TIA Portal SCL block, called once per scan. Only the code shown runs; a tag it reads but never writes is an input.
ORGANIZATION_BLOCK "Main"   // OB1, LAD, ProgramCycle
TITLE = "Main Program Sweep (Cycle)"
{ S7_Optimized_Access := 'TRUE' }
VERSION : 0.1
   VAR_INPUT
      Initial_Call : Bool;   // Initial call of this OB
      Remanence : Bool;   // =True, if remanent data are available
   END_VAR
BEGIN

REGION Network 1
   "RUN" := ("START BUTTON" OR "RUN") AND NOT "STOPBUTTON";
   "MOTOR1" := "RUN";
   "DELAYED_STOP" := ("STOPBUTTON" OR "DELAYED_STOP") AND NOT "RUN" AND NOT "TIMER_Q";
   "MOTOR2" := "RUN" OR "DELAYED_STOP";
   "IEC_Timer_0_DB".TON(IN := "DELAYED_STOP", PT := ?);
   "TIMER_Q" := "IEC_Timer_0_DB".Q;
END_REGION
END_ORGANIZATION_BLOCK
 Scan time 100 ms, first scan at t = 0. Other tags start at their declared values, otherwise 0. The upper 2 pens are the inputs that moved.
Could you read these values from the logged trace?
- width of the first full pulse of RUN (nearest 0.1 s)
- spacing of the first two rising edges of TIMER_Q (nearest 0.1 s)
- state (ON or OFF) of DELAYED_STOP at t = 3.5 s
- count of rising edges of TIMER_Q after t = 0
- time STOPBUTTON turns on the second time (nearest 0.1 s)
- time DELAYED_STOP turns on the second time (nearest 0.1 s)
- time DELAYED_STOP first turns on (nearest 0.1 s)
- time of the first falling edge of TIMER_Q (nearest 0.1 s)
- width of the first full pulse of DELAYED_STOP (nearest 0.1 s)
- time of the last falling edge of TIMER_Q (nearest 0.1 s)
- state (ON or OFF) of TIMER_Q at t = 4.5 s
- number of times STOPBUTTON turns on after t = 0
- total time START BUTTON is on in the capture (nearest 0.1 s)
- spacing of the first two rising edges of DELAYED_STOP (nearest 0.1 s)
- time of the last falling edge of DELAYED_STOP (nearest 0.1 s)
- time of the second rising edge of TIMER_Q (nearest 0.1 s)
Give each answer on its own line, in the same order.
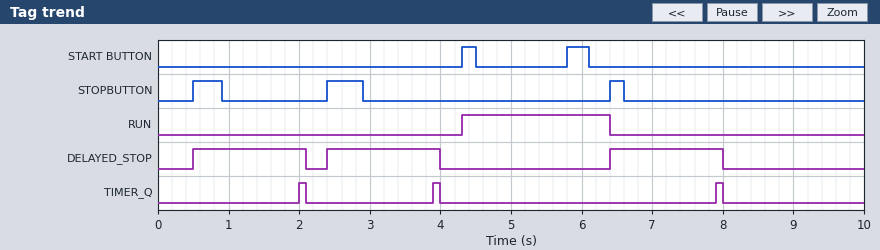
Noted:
2.1 s
1.9 s
ON
3
2.4 s
2.4 s
0.5 s
2.1 s
1.6 s
8.0 s
OFF
3
0.5 s
1.9 s
8.0 s
3.9 s
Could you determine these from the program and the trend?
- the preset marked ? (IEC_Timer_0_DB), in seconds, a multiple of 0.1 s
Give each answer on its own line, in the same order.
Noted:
1.5 s
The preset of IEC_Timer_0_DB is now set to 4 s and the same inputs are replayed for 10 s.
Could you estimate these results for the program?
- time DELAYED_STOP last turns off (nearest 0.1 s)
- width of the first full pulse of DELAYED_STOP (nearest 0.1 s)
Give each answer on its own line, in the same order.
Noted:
4.3 s
3.8 s
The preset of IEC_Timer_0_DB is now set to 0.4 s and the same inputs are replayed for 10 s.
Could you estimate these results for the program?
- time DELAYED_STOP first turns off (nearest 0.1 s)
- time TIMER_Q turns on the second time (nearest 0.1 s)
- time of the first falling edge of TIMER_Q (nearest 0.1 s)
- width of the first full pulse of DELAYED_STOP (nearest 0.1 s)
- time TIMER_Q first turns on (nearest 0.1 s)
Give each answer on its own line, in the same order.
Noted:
1.0 s
2.8 s
1.0 s
0.5 s
0.9 s
